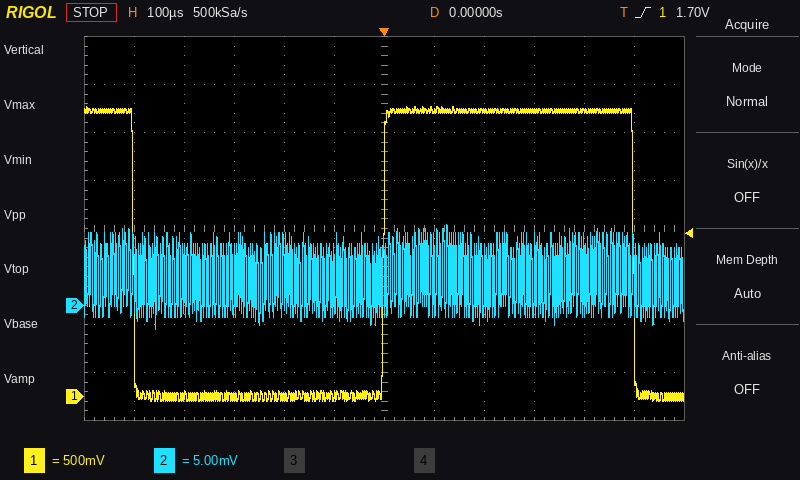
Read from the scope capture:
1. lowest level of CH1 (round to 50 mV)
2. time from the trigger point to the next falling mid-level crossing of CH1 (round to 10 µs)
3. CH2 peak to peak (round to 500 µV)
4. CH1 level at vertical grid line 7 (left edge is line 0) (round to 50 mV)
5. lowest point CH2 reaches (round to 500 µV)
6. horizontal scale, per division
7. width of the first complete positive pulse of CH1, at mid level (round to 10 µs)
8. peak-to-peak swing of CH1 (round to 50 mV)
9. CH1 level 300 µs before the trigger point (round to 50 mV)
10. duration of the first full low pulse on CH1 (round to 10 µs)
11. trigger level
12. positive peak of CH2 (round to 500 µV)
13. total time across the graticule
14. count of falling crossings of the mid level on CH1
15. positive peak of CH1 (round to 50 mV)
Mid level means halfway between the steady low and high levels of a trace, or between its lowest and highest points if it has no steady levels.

-50 mV
500 µs
11.0 mV
3.00 V
-2.5 mV
100 µs
500 µs
3.05 V
0 mV
500 µs
1.70 V
8.5 mV
1.2 ms
2
3.00 V
